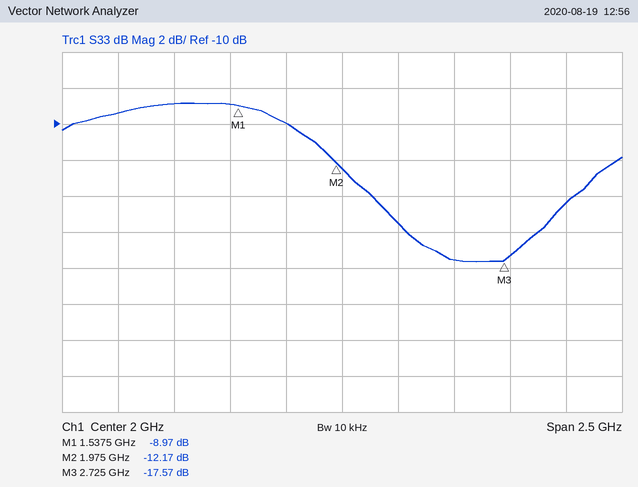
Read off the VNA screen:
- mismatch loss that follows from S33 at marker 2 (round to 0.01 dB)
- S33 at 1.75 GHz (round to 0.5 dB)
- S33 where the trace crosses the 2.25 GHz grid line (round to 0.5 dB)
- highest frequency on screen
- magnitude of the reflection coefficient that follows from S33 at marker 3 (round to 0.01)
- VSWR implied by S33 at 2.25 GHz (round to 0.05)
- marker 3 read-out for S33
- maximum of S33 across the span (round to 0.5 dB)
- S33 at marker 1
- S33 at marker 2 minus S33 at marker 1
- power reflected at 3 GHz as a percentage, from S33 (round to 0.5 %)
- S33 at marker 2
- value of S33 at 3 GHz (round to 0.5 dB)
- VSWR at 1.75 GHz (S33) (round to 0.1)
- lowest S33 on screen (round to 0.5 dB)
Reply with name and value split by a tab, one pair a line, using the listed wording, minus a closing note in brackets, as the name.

mismatch loss that follows from S33 at marker 2	0.27 dB
S33 at 1.75 GHz	-10.0 dB
S33 where the trace crosses the 2.25 GHz grid line	-15.5 dB
highest frequency on screen	3.25 GHz
magnitude of the reflection coefficient that follows from S33 at marker 3	0.13
VSWR implied by S33 at 2.25 GHz	1.40
marker 3 read-out for S33	-17.57 dB
maximum of S33 across the span	-9.0 dB
S33 at marker 1	-8.97 dB
S33 at marker 2 minus S33 at marker 1	-3.20 dB
power reflected at 3 GHz as a percentage, from S33	3.5 %
S33 at marker 2	-12.17 dB
value of S33 at 3 GHz	-14.5 dB
VSWR at 1.75 GHz (S33)	1.9
lowest S33 on screen	-17.5 dB
